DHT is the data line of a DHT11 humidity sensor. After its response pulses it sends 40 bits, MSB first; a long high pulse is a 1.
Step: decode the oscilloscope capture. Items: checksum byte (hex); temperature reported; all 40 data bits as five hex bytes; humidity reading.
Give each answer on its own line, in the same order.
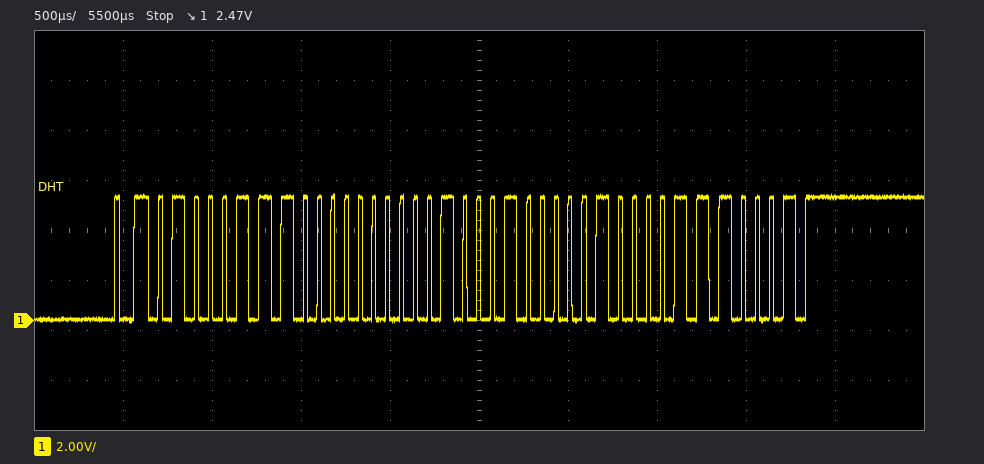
0x71
34.8 °C
47 00 22 08 71
71 %
